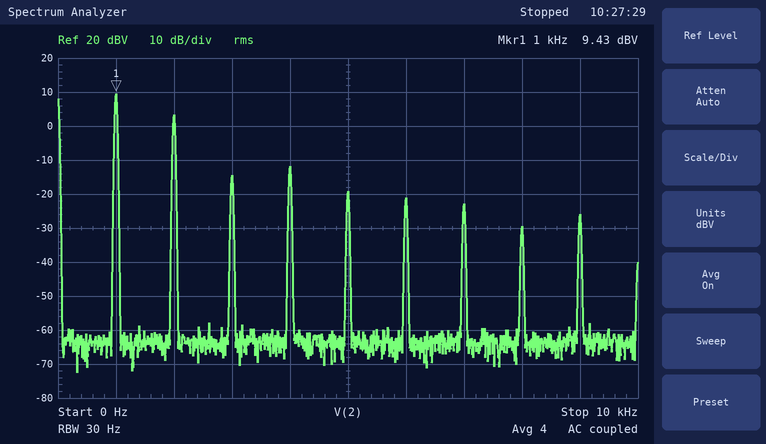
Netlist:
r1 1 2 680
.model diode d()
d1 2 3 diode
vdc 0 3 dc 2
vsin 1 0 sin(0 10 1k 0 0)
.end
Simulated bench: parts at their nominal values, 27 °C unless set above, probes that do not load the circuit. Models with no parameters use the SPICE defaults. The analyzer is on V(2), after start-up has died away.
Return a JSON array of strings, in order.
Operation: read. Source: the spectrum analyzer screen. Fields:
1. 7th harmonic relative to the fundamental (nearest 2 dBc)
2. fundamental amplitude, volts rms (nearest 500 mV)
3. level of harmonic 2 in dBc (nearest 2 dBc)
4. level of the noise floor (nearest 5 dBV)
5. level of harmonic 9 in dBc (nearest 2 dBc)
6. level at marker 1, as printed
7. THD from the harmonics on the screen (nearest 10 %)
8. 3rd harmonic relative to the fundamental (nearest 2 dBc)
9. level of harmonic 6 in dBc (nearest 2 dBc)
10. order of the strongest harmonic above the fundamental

["-32 dBc", "3.0 V", "-6 dBc", "-65 dBV", "-36 dBc", "9.43 dBV", "50 %", "-24 dBc", "-30 dBc", "2"]
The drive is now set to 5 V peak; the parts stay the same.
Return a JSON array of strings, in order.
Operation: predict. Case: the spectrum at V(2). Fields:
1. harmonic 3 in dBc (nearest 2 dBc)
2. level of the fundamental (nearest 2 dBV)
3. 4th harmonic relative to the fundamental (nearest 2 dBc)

["-16 dBc", "2 dBV", "-24 dBc"]
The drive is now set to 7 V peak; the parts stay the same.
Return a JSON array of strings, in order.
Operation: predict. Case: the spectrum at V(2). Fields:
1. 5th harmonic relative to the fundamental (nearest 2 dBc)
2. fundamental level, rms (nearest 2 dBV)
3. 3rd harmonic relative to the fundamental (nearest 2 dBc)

["-26 dBc", "6 dBV", "-20 dBc"]
